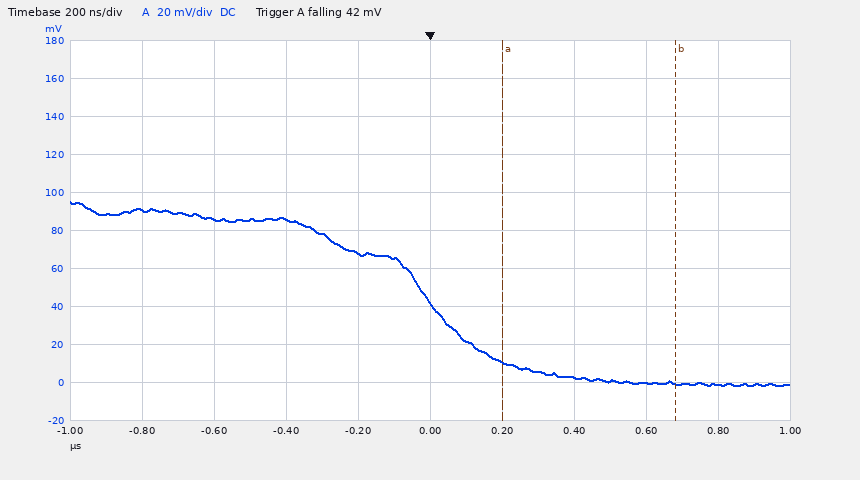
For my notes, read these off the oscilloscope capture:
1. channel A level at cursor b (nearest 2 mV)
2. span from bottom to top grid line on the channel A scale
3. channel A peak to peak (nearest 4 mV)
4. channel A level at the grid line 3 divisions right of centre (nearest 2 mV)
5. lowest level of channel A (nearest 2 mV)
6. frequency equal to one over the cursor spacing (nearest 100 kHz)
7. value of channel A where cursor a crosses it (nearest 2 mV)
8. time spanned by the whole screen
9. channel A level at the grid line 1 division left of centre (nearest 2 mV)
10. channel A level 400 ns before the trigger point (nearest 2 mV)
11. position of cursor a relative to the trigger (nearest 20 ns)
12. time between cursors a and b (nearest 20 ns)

0 mV
200 mV
96 mV
0 mV
-2 mV
2.1 MHz
10 mV
2 µs
68 mV
86 mV
+200 ns
480 ns
